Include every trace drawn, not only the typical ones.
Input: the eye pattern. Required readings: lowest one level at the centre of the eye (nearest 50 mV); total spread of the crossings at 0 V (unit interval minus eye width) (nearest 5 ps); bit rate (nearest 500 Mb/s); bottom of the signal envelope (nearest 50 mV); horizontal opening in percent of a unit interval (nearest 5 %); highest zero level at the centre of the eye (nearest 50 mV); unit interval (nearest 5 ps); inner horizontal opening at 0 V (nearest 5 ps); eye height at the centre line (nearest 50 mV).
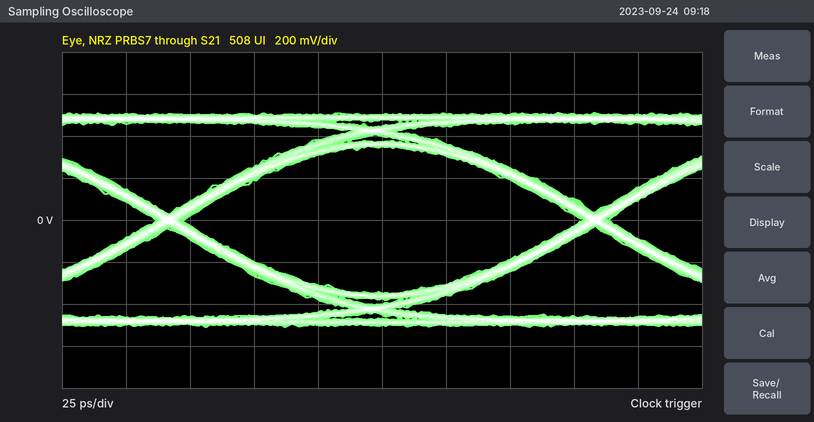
350 mV
10 ps
6.0 Gb/s
-500 mV
95 %
-350 mV
165 ps
155 ps
700 mV
